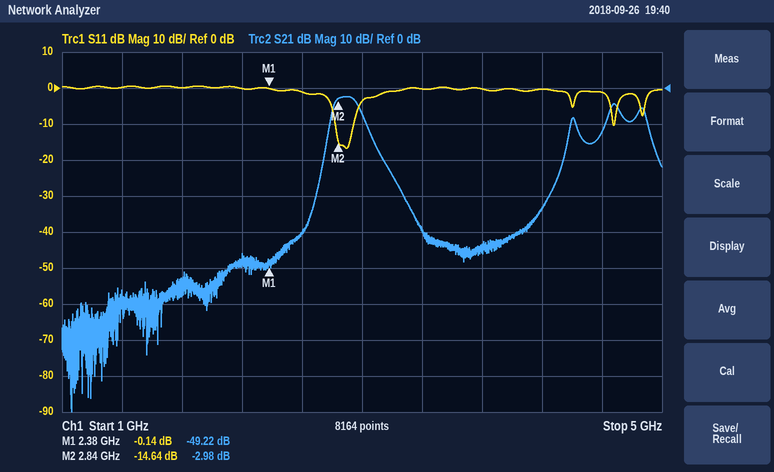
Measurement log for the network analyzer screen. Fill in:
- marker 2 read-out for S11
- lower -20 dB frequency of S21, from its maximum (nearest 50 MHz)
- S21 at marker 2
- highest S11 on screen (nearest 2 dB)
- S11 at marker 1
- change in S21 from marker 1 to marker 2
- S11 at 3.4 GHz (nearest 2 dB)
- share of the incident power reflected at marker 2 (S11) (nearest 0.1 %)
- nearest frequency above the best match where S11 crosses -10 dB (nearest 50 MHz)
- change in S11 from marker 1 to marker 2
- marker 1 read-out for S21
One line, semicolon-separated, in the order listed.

-14.64 dB; 2.75 GHz; -2.98 dB; 0 dB; -0.14 dB; 46.24 dB; 0 dB; 3.4 %; 2.95 GHz; -14.50 dB; -49.22 dB
